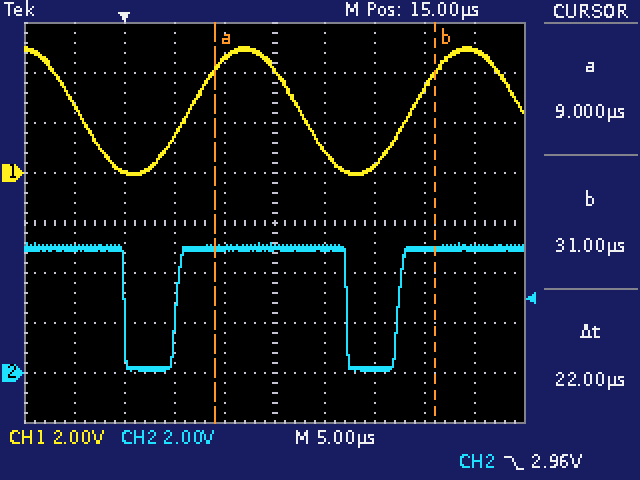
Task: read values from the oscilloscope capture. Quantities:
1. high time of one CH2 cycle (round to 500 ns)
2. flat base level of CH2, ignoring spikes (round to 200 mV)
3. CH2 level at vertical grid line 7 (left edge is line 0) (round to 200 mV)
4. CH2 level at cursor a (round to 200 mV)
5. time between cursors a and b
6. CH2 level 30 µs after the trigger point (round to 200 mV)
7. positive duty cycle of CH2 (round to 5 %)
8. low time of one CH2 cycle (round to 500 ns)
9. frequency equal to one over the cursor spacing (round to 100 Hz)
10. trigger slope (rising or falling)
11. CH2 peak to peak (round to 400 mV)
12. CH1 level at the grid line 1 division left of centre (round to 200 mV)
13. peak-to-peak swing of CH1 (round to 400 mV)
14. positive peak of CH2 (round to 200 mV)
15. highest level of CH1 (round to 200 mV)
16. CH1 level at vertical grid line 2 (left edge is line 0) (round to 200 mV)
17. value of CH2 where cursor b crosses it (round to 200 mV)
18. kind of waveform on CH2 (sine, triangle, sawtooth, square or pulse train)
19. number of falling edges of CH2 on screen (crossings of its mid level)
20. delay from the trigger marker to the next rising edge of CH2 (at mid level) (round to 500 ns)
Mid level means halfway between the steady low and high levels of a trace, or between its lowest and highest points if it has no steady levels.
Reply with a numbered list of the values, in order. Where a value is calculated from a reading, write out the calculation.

1. 17.0 µs
2. 200 mV
3. 200 mV
4. 5.0 V
5. 22 µs
6. 5.0 V
7. 75 %
8. 5.0 µs
9. 1 / 22 µs ≈ 45.5 kHz
10. falling
11. 5.2 V
12. 4.6 V
13. 5.2 V
14. 5.2 V
15. 5.0 V
16. 0.0 V
17. 5.0 V
18. pulse train
19. 2
20. 5.0 µs
